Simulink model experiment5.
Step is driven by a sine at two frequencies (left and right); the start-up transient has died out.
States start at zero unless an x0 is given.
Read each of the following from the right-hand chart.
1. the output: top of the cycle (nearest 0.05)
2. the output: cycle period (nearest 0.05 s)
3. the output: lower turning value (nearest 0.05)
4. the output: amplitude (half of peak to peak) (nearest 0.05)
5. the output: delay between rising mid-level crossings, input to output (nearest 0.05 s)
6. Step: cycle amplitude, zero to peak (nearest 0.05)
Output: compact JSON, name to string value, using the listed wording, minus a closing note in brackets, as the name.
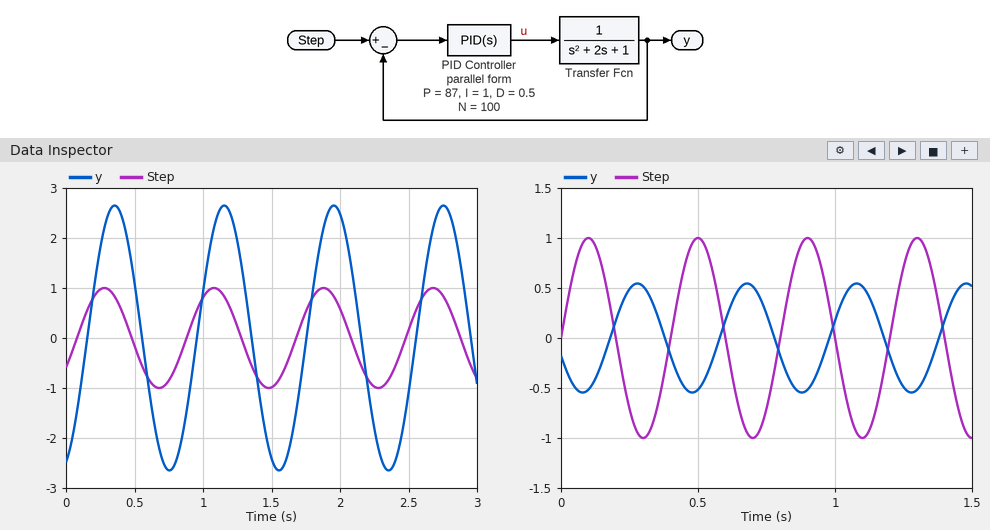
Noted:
{"the output: top of the cycle": "0.55", "the output: cycle period": "0.40 s", "the output: lower turning value": "-0.55", "the output: amplitude (half of peak to peak)": "0.55", "the output: delay between rising mid-level crossings, input to output": "0.20 s", "Step: cycle amplitude, zero to peak": "1.00"}
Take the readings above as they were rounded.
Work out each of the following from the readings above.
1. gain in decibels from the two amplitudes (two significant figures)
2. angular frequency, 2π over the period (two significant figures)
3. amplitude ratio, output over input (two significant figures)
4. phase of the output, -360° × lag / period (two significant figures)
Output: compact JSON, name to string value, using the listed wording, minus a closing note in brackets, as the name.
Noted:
{"gain in decibels from the two amplitudes": "-5.2 dB", "angular frequency, 2π over the period": "16 rad/s", "amplitude ratio, output over input": "0.55", "phase of the output, -360° × lag / period": "-180°"}
